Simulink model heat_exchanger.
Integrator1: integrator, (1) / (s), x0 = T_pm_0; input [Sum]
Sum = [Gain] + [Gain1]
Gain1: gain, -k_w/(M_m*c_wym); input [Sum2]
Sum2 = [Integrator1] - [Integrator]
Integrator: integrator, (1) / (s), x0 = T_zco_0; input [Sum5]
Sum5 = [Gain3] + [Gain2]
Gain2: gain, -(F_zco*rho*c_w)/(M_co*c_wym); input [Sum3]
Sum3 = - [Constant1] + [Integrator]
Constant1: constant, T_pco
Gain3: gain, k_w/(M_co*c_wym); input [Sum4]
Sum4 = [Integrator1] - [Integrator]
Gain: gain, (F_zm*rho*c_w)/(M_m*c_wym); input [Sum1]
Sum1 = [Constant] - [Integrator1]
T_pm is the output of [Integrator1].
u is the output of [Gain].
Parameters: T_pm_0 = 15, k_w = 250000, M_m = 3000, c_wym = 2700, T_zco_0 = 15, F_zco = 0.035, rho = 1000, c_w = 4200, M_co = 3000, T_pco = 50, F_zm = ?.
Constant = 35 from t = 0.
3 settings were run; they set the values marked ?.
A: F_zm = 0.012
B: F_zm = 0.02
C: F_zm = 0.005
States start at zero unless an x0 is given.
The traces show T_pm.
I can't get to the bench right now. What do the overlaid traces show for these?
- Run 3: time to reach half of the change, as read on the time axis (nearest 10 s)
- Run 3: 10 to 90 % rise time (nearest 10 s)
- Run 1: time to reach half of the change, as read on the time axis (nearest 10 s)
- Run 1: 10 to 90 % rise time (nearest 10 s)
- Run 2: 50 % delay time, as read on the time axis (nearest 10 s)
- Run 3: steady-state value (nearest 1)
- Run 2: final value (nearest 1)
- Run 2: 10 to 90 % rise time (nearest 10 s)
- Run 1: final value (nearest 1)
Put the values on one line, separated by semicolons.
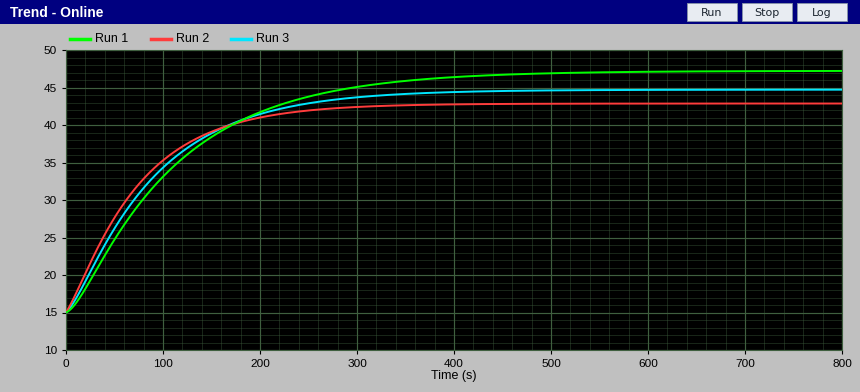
70 s; 190 s; 90 s; 240 s; 60 s; 45; 43; 160 s; 47
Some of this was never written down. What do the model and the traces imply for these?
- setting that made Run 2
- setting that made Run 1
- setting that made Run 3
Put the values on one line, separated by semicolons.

B; C; A
